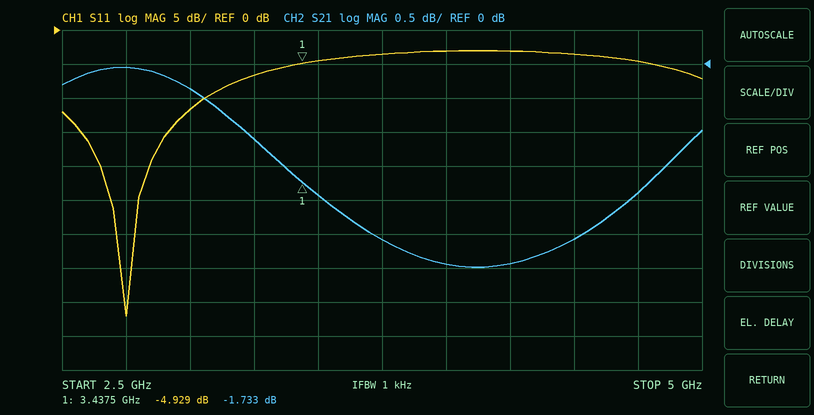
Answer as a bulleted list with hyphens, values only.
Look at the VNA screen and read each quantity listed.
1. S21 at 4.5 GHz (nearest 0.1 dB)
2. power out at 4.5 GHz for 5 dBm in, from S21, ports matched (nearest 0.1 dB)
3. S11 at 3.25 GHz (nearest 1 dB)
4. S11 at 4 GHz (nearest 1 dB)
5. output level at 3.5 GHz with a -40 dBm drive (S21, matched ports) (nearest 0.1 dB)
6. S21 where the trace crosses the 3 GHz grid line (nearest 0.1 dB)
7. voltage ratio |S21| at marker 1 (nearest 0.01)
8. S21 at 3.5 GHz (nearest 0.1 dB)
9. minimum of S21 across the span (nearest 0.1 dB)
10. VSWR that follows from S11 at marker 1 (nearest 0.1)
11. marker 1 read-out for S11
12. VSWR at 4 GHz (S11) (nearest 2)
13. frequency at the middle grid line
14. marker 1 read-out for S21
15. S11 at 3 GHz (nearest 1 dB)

- -2.6 dB
- 2.4 dBm
- -7 dB
- -3 dB
- -41.9 dBm
- -0.4 dB
- 0.82
- -1.9 dB
- -3.0 dB
- 3.6
- -4.929 dB
- 6
- 3.75 GHz
- -1.733 dB
- -12 dB
